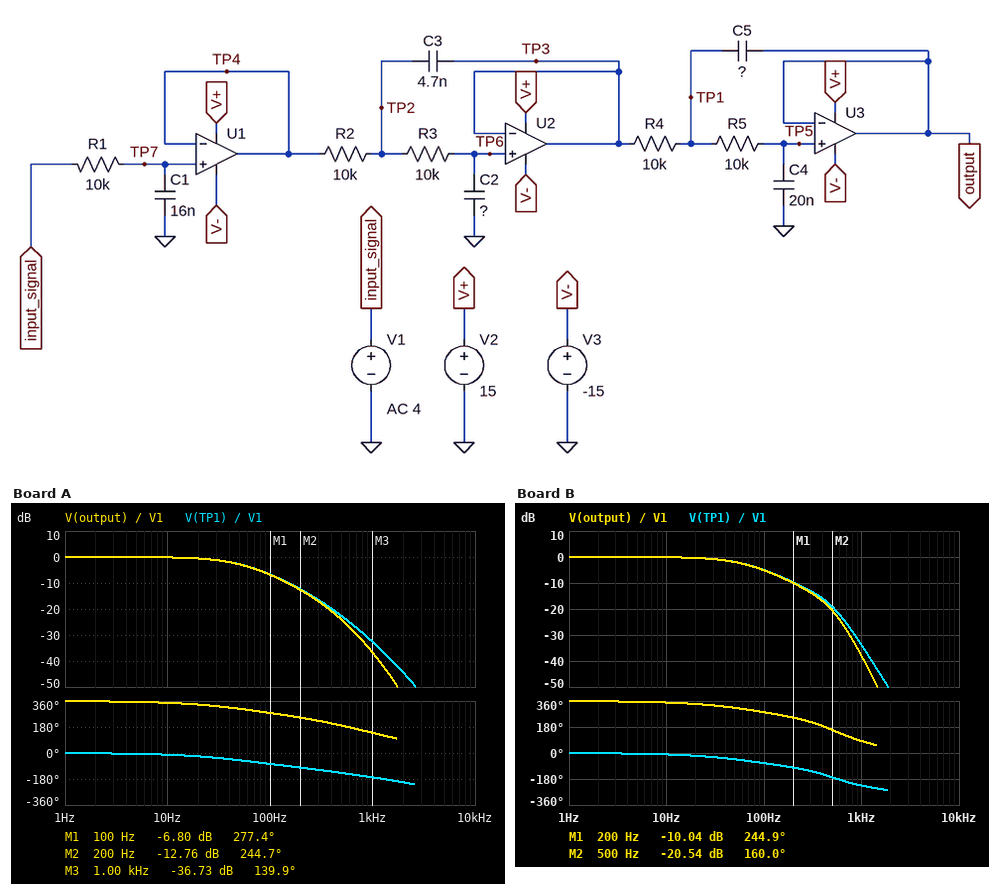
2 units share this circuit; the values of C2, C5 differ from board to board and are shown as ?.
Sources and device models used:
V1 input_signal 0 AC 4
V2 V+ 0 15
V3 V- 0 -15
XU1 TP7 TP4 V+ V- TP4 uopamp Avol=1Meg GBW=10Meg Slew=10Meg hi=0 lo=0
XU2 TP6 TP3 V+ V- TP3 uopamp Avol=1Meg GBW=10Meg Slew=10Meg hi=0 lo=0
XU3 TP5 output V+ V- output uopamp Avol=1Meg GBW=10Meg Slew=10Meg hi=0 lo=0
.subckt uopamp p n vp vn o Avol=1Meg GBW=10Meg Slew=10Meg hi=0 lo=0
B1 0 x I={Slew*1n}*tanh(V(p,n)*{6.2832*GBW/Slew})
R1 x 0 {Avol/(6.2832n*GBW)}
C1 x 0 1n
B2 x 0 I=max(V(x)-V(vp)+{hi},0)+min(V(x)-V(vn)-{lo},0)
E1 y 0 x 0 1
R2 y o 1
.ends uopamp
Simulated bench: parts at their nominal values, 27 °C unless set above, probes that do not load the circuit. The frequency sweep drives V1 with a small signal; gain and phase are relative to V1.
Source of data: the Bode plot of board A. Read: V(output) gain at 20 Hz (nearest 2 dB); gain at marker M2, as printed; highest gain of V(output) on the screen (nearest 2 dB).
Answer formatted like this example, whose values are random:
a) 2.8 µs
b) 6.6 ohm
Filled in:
a) 0 dB
b) -12.76 dB
c) 0 dB
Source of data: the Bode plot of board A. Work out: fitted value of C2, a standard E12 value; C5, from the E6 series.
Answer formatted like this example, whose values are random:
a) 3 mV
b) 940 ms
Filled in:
a) 150 nF
b) 6.8 nF
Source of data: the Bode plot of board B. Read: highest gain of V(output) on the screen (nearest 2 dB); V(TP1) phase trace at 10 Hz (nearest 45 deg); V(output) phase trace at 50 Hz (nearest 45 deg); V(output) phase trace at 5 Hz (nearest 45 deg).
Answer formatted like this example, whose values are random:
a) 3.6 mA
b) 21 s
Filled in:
a) 0 dB
b) 0 deg
c) 315 deg
d) 360 deg
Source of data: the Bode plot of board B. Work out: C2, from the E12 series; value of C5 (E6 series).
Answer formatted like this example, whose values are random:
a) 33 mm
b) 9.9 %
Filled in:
a) 120 nF
b) 47 nF
